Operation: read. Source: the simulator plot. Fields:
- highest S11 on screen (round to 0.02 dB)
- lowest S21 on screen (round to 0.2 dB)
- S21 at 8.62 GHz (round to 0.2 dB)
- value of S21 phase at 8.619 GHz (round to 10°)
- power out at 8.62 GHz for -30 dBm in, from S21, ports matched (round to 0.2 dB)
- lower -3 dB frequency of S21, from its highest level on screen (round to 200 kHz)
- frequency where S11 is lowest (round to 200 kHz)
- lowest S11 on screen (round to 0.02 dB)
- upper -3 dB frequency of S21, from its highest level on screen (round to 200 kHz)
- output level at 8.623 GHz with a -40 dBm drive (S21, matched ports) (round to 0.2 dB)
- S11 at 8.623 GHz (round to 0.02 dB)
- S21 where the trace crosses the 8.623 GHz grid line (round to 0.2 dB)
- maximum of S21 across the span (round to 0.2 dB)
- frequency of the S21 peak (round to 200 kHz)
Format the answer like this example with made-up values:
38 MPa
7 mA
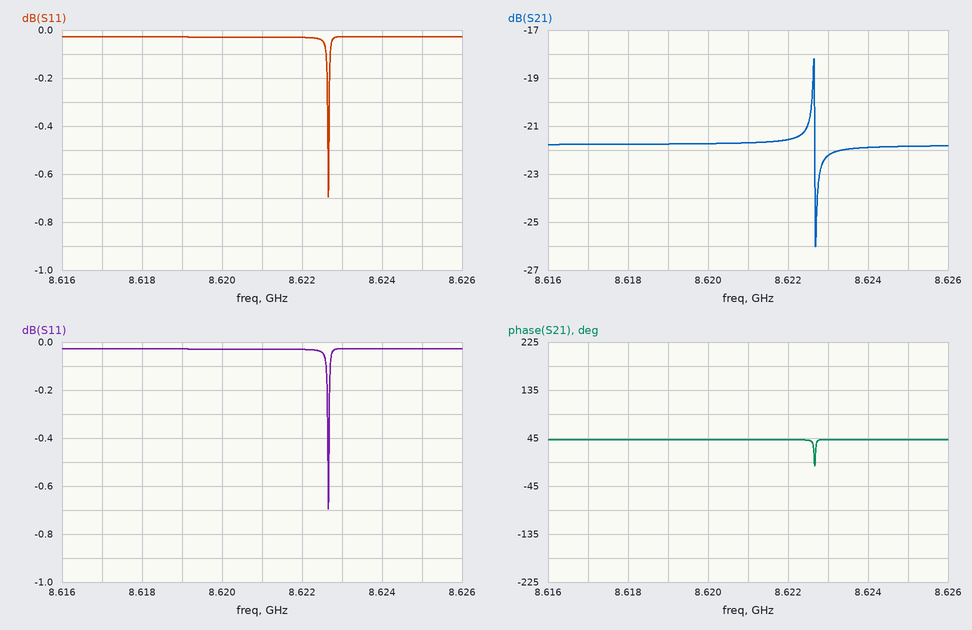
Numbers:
-0.02 dB
-26.0 dB
-21.8 dB
40°
-51.8 dBm
8.6224 GHz
8.6226 GHz
-0.70 dB
8.6226 GHz
-62.2 dBm
-0.02 dB
-22.2 dB
-18.2 dB
8.6226 GHz
